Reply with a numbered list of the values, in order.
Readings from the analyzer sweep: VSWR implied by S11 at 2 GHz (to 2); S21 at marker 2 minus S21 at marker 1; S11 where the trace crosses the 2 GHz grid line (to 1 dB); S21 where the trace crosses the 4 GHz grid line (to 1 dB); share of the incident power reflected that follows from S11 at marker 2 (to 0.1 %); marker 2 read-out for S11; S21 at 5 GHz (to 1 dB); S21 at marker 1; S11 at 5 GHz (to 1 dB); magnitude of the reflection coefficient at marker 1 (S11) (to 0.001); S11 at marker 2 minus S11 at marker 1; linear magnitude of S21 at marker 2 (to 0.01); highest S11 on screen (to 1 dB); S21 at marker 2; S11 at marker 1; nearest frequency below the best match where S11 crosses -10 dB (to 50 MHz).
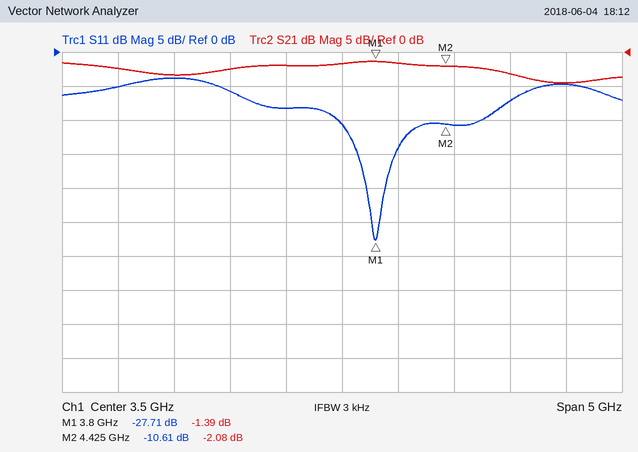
1. 4
2. -0.69 dB
3. -4 dB
4. -2 dB
5. 8.7 %
6. -10.61 dB
7. -3 dB
8. -1.39 dB
9. -7 dB
10. 0.041
11. 17.10 dB
12. 0.79
13. -4 dB
14. -2.08 dB
15. -27.71 dB
16. 3.45 GHz
